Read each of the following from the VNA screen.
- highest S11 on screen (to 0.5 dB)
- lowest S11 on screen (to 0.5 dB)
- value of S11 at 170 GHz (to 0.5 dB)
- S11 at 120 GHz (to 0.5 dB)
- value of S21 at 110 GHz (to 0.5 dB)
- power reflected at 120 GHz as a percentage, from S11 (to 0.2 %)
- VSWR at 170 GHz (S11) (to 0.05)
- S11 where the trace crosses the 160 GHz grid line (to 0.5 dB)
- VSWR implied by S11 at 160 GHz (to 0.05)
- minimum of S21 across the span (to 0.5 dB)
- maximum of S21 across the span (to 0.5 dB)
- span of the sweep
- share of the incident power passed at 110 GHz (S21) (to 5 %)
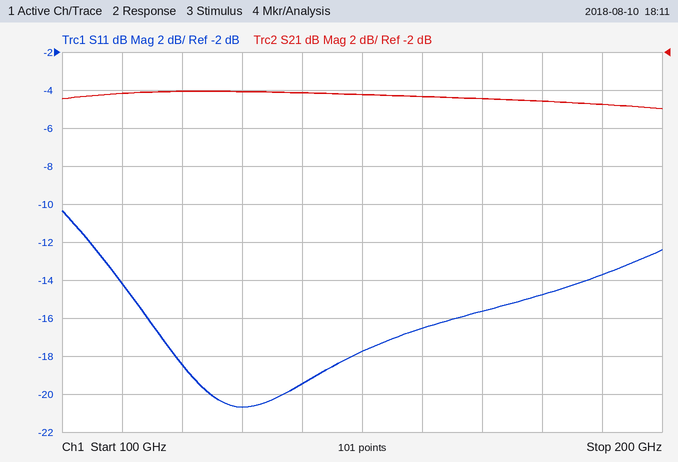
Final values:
-10.5 dB
-20.5 dB
-15.5 dB
-18.5 dB
-4.0 dB
1.4 %
1.40
-16.5 dB
1.35
-5.0 dB
-4.0 dB
100 GHz
40 %
